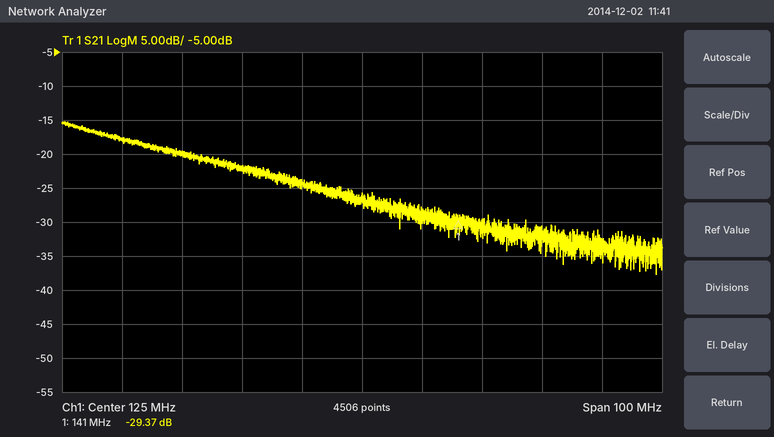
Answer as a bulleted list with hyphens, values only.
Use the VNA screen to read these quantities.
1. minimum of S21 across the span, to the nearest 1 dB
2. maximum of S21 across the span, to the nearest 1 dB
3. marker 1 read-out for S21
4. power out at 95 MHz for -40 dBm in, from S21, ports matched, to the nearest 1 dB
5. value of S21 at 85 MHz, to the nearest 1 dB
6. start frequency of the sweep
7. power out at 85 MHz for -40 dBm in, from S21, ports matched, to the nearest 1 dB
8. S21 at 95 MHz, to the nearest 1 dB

- -38 dB
- -15 dB
- -29.37 dB
- -60 dBm
- -18 dB
- 75 MHz
- -58 dBm
- -20 dB
